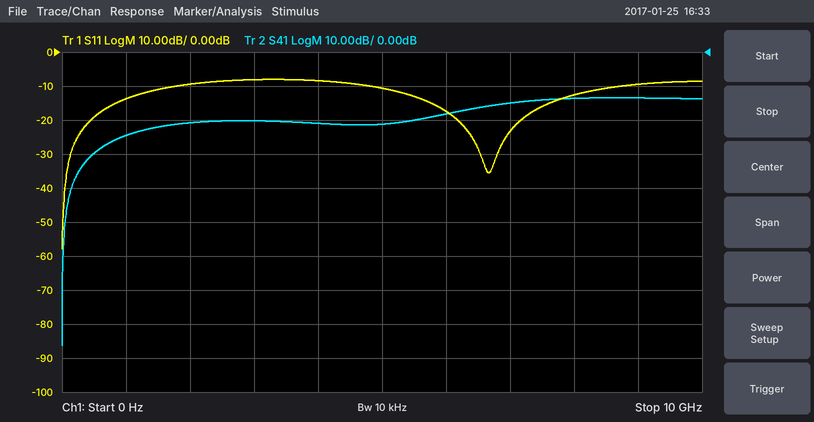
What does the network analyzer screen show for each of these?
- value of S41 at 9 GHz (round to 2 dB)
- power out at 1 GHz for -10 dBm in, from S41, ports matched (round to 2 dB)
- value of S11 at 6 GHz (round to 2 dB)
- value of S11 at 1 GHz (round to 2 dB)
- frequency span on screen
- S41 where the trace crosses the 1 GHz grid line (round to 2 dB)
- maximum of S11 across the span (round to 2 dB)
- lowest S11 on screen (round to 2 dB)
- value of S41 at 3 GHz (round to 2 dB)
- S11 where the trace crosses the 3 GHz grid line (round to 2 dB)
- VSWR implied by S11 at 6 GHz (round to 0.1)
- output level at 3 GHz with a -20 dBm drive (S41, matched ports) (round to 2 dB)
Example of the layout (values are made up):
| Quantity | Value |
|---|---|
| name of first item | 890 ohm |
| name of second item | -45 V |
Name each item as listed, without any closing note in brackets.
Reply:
| Quantity | Value |
|---|---|
| value of S41 at 9 GHz | -14 dB |
| power out at 1 GHz for -10 dBm in, from S41, ports matched | -34 dBm |
| value of S11 at 6 GHz | -18 dB |
| value of S11 at 1 GHz | -14 dB |
| frequency span on screen | 10 GHz |
| S41 where the trace crosses the 1 GHz grid line | -24 dB |
| maximum of S11 across the span | -8 dB |
| lowest S11 on screen | -58 dB |
| value of S41 at 3 GHz | -20 dB |
| S11 where the trace crosses the 3 GHz grid line | -8 dB |
| VSWR implied by S11 at 6 GHz | 1.3 |
| output level at 3 GHz with a -20 dBm drive (S41, matched ports) | -40 dBm |
